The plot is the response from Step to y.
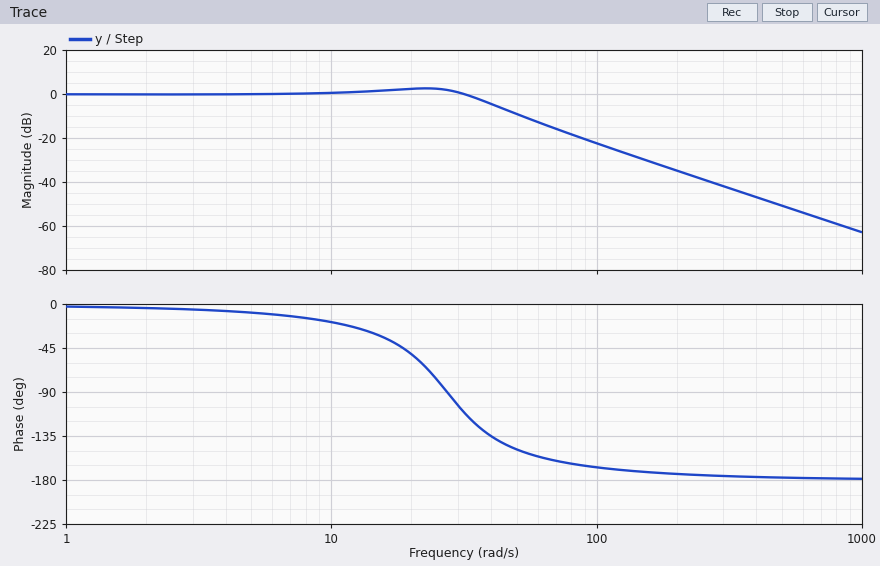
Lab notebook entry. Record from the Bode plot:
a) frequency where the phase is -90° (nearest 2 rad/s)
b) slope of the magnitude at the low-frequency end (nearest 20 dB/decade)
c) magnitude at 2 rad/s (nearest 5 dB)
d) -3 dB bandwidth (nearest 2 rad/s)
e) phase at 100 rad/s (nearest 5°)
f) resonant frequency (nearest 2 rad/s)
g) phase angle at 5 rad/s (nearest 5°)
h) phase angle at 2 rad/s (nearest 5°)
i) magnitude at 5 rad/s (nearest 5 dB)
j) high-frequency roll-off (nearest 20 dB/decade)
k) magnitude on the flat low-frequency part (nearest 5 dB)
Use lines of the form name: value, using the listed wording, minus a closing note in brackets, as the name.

frequency where the phase is -90°: 28 rad/s
slope of the magnitude at the low-frequency end: 0 dB/decade
magnitude at 2 rad/s: 0 dB
-3 dB bandwidth: 38 rad/s
phase at 100 rad/s: -165°
resonant frequency: 22 rad/s
phase angle at 5 rad/s: -10°
phase angle at 2 rad/s: -5°
magnitude at 5 rad/s: 0 dB
high-frequency roll-off: -40 dB/decade
magnitude on the flat low-frequency part: 0 dB
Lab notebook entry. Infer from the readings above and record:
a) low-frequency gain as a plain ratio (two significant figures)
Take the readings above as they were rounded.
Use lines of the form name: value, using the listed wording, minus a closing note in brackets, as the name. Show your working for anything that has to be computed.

low-frequency gain as a plain ratio: 10^(0 / 20) = 1.0
